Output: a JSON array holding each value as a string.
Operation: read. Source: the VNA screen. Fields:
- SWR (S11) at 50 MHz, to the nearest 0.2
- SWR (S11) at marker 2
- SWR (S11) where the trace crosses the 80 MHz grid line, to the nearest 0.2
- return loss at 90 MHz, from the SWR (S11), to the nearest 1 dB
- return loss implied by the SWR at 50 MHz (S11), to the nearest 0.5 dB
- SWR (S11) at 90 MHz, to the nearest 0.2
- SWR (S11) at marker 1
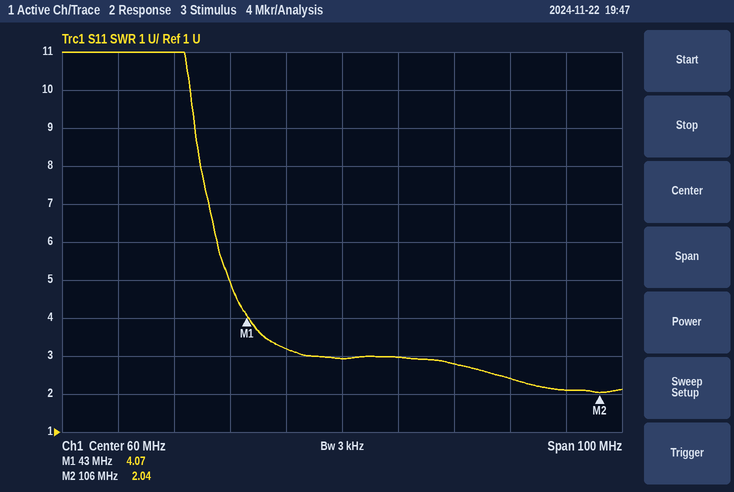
["3.2", "2.04", "2.8", "8 dB", "5.5 dB", "2.4", "4.07"]
